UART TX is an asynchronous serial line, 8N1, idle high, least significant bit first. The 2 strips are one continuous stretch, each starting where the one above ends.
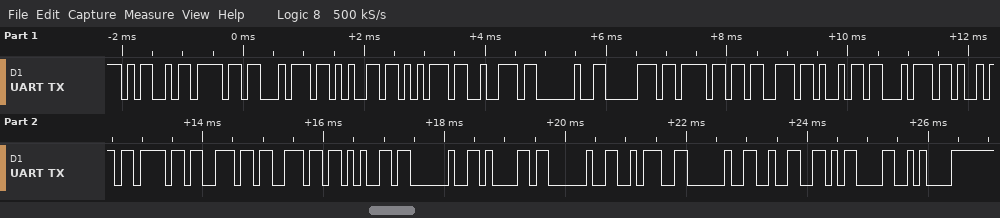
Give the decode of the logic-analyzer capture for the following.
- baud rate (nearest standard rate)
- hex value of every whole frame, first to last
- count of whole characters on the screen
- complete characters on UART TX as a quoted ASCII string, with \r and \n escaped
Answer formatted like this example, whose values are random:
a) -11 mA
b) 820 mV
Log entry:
a) 9600 baud
b) 4D 6F 74 65 75 72 20 70 6F 73 69 74 69 6F 6E 6E 65 20 61 20 3A 20 32 0D 0A
c) 25
d) "Moteur positionne a : 2\r\n"
